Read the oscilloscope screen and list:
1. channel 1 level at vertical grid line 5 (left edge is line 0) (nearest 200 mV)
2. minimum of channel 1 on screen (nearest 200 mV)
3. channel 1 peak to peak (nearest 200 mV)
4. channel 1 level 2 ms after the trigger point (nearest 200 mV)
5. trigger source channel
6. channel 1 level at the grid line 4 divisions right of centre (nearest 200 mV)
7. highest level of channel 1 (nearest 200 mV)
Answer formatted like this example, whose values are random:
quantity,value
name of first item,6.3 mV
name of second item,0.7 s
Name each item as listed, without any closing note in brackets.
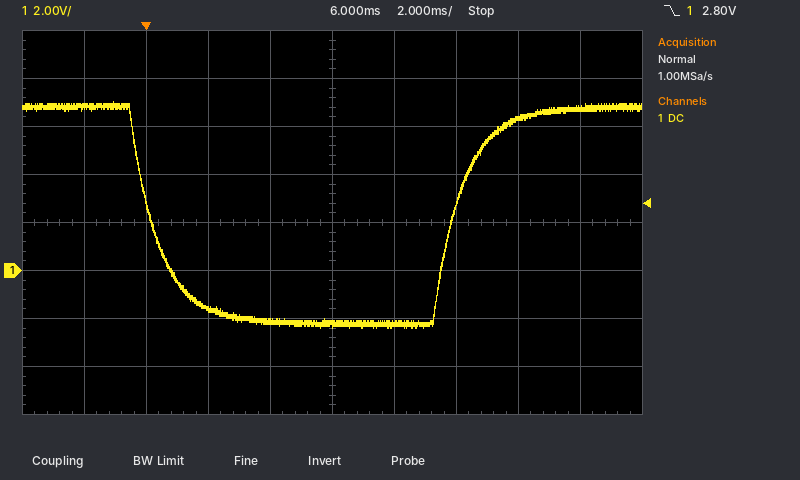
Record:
quantity,value
channel 1 level at vertical grid line 5 (left edge is line 0),-2.2 V
minimum of channel 1 on screen,-2.4 V
channel 1 peak to peak,9.4 V
channel 1 level 2 ms after the trigger point,-1.6 V
trigger source channel,channel 1
channel 1 level at the grid line 4 divisions right of centre,6.8 V
highest level of channel 1,7.0 V
